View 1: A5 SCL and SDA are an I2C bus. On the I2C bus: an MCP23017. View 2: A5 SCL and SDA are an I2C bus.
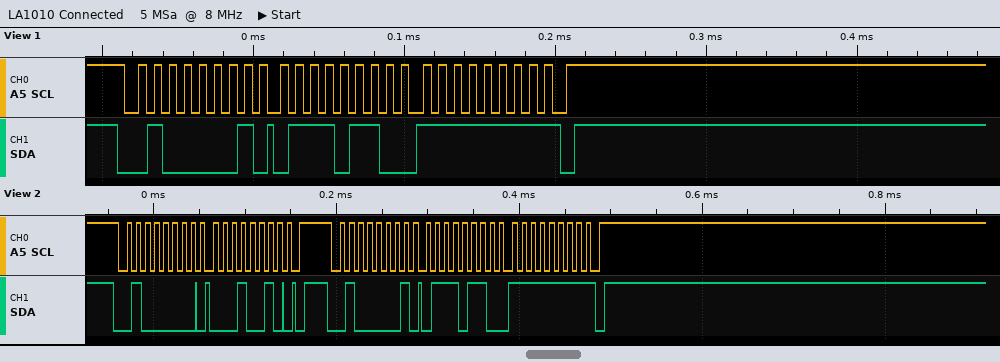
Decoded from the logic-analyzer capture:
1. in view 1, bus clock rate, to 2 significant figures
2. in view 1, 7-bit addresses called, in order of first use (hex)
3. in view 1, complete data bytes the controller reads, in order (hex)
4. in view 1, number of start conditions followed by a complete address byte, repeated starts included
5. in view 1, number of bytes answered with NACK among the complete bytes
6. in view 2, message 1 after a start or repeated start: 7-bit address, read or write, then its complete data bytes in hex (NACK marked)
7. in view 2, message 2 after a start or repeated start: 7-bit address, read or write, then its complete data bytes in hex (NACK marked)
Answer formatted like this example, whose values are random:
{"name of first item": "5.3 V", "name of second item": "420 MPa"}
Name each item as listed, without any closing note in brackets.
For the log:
{"in view 1, bus clock rate, to 2 significant figures": "100 kHz", "in view 1, 7-bit addresses called, in order of first use": "0x20", "in view 1, complete data bytes the controller reads, in order": "76 FF", "in view 1, number of start conditions followed by a complete address byte, repeated starts included": "1", "in view 1, number of bytes answered with NACK among the complete bytes": "1", "in view 2, message 1 after a start or repeated start: 7-bit address, read or write, then its complete data bytes in hex": "0x20 write: 12", "in view 2, message 2 after a start or repeated start: 7-bit address, read or write, then its complete data bytes in hex": "0x20 read: 76 FF NACK"}
